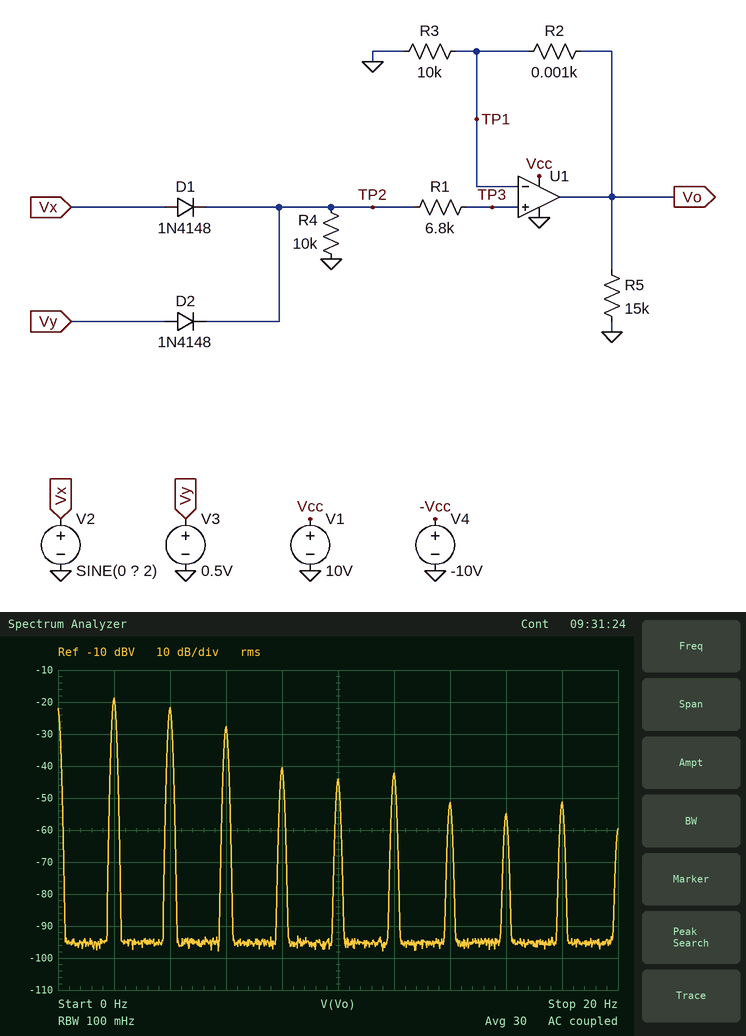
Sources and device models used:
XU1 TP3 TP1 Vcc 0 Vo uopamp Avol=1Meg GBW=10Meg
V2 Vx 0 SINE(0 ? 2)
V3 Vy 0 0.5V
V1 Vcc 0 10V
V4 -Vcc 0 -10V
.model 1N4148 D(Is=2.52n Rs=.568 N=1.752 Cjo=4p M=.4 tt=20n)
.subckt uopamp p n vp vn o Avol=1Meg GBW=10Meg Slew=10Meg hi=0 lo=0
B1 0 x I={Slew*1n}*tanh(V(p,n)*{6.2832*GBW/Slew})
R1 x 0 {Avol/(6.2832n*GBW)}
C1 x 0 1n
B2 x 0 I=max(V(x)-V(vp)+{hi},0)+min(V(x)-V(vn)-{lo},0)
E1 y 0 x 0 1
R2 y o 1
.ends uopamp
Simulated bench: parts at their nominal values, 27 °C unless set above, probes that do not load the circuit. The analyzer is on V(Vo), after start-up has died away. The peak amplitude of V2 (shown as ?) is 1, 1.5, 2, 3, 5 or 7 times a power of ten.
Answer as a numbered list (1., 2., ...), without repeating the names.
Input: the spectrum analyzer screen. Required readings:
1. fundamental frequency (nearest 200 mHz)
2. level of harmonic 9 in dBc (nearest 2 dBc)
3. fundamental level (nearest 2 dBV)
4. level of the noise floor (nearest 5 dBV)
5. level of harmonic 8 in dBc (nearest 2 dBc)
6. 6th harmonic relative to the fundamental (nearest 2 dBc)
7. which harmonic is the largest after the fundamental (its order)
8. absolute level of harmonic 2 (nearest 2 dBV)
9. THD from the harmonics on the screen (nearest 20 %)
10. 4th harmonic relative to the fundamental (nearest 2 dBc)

1. 2.0 Hz
2. -32 dBc
3. -18 dBV
4. -95 dBV
5. -36 dBc
6. -24 dBc
7. 2
8. -22 dBV
9. 80 %
10. -22 dBc
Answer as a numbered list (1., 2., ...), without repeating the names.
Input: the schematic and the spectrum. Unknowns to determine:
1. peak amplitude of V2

1. 1 V
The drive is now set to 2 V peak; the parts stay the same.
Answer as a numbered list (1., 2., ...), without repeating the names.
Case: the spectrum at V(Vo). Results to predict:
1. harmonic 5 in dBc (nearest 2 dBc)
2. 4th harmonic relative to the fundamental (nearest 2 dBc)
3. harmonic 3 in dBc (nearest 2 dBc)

1. -24 dBc
2. -24 dBc
3. -16 dBc
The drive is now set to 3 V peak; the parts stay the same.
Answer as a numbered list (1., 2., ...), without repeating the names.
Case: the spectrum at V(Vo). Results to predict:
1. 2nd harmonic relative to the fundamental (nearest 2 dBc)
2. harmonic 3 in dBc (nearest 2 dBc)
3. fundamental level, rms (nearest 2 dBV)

1. -6 dBc
2. -20 dBc
3. -2 dBV
